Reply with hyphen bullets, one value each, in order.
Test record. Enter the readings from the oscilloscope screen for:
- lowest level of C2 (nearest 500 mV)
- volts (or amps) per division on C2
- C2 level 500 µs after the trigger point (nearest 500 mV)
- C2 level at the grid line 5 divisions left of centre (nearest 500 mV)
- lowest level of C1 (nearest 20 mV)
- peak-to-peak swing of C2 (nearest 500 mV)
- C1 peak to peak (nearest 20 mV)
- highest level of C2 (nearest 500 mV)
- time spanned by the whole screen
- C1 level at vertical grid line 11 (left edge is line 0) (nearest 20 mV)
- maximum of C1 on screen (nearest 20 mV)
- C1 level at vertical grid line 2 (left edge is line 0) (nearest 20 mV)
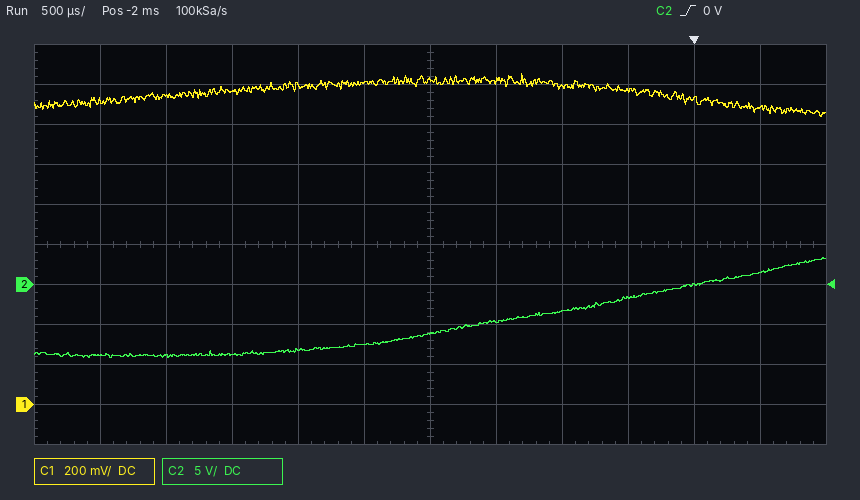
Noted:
- -9.0 V
- 5 V
- 1.5 V
- -9.0 V
- 1.44 V
- 12.5 V
- 220 mV
- 3.5 V
- 6 ms
- 1.48 V
- 1.66 V
- 1.54 V
